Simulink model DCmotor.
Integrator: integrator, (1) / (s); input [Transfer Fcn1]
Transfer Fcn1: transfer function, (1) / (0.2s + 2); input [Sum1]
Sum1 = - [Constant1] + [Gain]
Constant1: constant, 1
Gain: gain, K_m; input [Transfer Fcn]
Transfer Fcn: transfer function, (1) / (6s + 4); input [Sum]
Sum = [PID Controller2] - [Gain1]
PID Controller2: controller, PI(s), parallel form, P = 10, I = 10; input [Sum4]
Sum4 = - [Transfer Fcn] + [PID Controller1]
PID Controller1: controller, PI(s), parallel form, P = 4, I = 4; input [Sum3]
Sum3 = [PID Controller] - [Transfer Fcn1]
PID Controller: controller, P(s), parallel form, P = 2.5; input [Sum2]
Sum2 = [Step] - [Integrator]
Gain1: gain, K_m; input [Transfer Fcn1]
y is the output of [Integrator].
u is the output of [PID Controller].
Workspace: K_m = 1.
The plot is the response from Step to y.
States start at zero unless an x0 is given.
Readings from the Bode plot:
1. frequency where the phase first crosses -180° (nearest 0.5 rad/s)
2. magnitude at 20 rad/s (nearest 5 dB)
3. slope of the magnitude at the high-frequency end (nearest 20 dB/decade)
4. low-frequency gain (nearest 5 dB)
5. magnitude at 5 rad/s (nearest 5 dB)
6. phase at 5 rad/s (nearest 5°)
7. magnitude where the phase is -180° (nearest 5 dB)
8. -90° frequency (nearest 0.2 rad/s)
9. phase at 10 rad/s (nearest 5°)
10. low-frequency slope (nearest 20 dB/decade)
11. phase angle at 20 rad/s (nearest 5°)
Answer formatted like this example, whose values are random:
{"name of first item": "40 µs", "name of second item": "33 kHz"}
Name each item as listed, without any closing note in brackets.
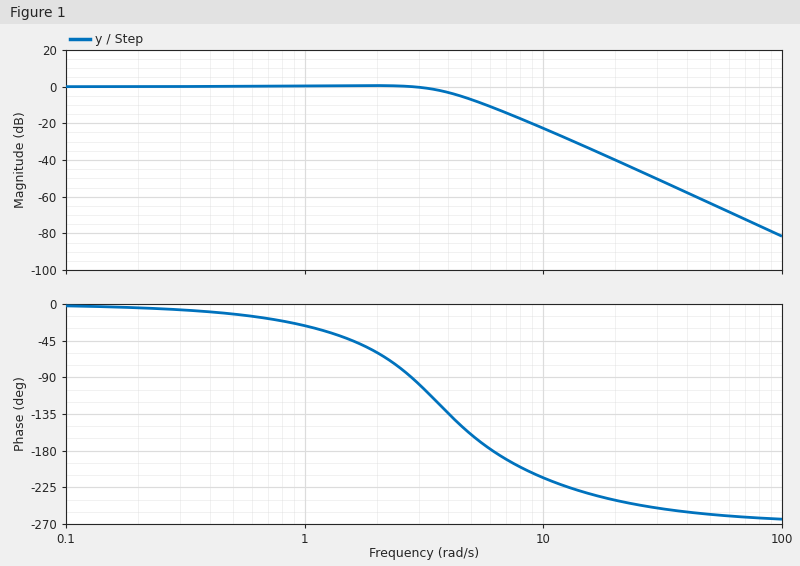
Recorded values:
{"frequency where the phase first crosses -180°": "6.0 rad/s", "magnitude at 20 rad/s": "-40 dB", "slope of the magnitude at the high-frequency end": "-60 dB/decade", "low-frequency gain": "0 dB", "magnitude at 5 rad/s": "-5 dB", "phase at 5 rad/s": "-160°", "magnitude where the phase is -180°": "-10 dB", "-90° frequency": "2.8 rad/s", "phase at 10 rad/s": "-215°", "low-frequency slope": "0 dB/decade", "phase angle at 20 rad/s": "-240°"}
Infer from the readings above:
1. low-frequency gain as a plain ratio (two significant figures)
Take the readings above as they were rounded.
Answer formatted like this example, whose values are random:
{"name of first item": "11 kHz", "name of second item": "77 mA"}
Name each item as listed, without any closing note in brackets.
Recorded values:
{"low-frequency gain as a plain ratio": "1.0"}
